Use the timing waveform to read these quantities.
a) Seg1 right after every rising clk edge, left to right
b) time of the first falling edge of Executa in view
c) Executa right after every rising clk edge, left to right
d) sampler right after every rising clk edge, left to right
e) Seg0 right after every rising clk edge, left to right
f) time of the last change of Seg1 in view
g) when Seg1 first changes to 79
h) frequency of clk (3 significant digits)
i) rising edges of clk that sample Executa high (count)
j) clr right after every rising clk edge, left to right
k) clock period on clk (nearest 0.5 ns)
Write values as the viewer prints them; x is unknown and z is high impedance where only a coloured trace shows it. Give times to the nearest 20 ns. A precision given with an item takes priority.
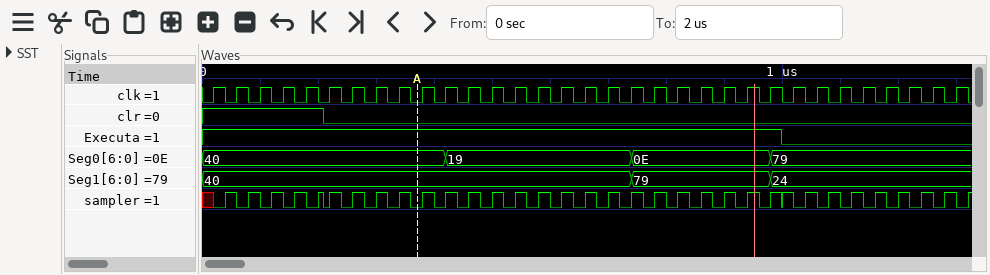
40, 40, 40, 40, 40, 40, 40, 40, 40, 40, 40, 40, 40, 40, 40, 40, 40, 40, 79, 79, 79, 79, 79, 79, 24, 24, 24, 24, 24, 24, 24, 24, 24
1000 ns
1 1 1 1 1 1 1 1 1 1 1 1 1 1 1 1 1 1 1 1 1 1 1 1 1 0 0 0 0 0 0 0 0
0 0 0 0 0 1 1 1 1 1 1 1 1 1 1 1 1 1 1 1 1 1 1 1 1 0 0 0 0 0 0 0 0
40, 40, 40, 40, 40, 40, 40, 40, 40, 40, 19, 19, 19, 19, 19, 19, 19, 19, 0E, 0E, 0E, 0E, 0E, 0E, 79, 79, 79, 79, 79, 79, 79, 79, 79
980 ns
740 ns
25.0 MHz
25
1 1 1 1 1 0 0 0 0 0 0 0 0 0 0 0 0 0 0 0 0 0 0 0 0 0 0 0 0 0 0 0 0
40 ns
